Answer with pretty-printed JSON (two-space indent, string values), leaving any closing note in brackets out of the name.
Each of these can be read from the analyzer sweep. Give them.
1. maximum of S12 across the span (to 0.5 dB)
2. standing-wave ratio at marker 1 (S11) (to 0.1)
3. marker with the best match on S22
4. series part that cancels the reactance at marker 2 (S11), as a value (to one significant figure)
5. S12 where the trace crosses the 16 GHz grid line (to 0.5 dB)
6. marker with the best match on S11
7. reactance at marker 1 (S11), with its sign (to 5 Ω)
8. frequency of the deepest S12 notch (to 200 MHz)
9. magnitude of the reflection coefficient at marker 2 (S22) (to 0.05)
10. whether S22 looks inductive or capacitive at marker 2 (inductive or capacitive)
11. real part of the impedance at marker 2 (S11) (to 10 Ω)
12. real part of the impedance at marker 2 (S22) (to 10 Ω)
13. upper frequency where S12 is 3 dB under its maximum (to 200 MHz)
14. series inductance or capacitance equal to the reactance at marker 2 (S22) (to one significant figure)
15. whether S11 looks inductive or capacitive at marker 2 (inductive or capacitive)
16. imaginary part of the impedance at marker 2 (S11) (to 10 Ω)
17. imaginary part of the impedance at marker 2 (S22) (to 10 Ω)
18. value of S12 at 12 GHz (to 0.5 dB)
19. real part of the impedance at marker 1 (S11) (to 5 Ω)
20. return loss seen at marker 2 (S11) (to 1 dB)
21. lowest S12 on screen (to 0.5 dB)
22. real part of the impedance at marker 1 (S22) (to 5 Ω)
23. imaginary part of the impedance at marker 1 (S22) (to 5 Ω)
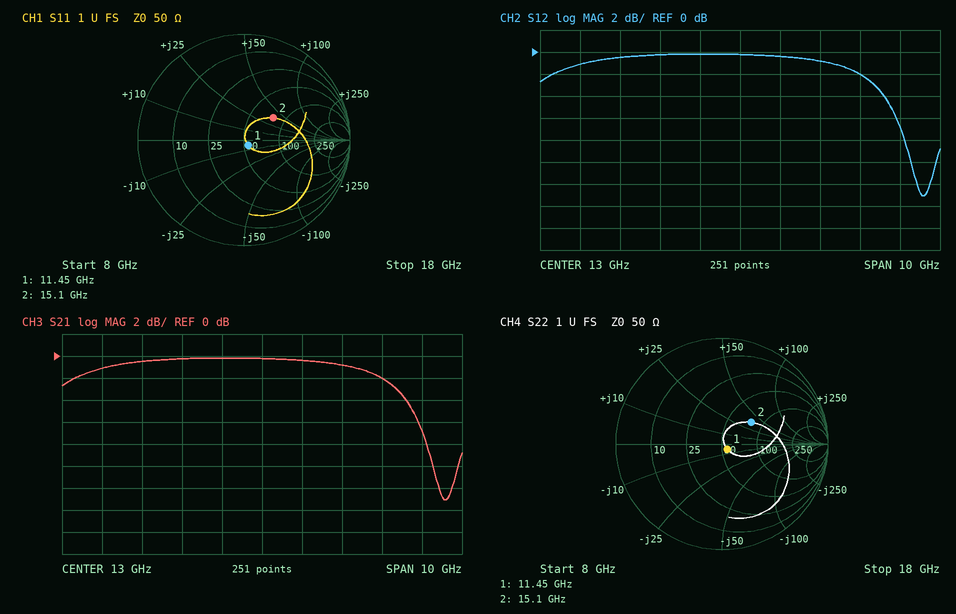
{
  "maximum of S12 across the span": "0.0 dB",
  "standing-wave ratio at marker 1 (S11)": "1.1",
  "marker with the best match on S22": "marker 1",
  "series part that cancels the reactance at marker 2 (S11), as a value": "300 fF",
  "S12 where the trace crosses the 16 GHz grid line": "-2.0 dB",
  "marker with the best match on S11": "marker 1",
  "reactance at marker 1 (S11), with its sign": "-5 Ω",
  "frequency of the deepest S12 notch": "17.6 GHz",
  "magnitude of the reflection coefficient at marker 2 (S22)": "0.35",
  "whether S22 looks inductive or capacitive at marker 2": "inductive",
  "real part of the impedance at marker 2 (S11)": "80 Ω",
  "real part of the impedance at marker 2 (S22)": "80 Ω",
  "upper frequency where S12 is 3 dB under its maximum": "16.4 GHz",
  "series inductance or capacitance equal to the reactance at marker 2 (S22)": "400 pH",
  "whether S11 looks inductive or capacitive at marker 2": "inductive",
  "imaginary part of the impedance at marker 2 (S11)": "+40 Ω",
  "imaginary part of the impedance at marker 2 (S22)": "+40 Ω",
  "value of S12 at 12 GHz": "0.0 dB",
  "real part of the impedance at marker 1 (S11)": "55 Ω",
  "return loss seen at marker 2 (S11)": "9 dB",
  "lowest S12 on screen": "-13.0 dB",
  "real part of the impedance at marker 1 (S22)": "55 Ω",
  "imaginary part of the impedance at marker 1 (S22)": "-5 Ω"
}
